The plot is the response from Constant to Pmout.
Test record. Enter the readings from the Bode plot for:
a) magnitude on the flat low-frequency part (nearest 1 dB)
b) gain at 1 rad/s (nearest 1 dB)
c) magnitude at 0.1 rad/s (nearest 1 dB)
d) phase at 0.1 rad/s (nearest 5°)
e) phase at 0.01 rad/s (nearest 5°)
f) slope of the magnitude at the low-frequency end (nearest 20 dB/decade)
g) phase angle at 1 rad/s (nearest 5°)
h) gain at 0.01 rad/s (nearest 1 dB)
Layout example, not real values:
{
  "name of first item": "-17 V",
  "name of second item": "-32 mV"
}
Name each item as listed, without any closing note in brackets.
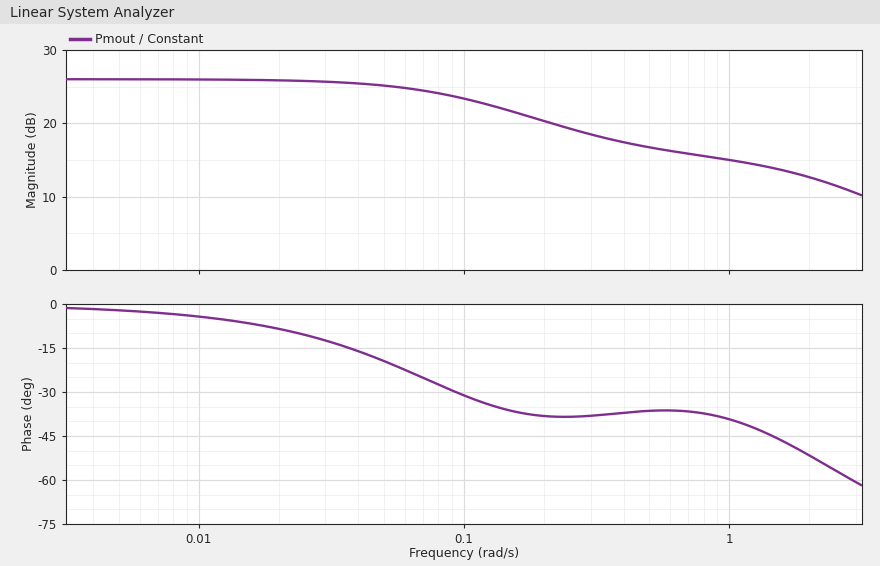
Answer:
{
  "magnitude on the flat low-frequency part": "26 dB",
  "gain at 1 rad/s": "15 dB",
  "magnitude at 0.1 rad/s": "23 dB",
  "phase at 0.1 rad/s": "-30°",
  "phase at 0.01 rad/s": "-5°",
  "slope of the magnitude at the low-frequency end": "0 dB/decade",
  "phase angle at 1 rad/s": "-40°",
  "gain at 0.01 rad/s": "26 dB"
}
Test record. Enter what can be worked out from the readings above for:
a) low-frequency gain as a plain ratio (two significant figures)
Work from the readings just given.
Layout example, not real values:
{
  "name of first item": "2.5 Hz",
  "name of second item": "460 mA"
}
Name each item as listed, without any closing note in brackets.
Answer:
{
  "low-frequency gain as a plain ratio": "20"
}
